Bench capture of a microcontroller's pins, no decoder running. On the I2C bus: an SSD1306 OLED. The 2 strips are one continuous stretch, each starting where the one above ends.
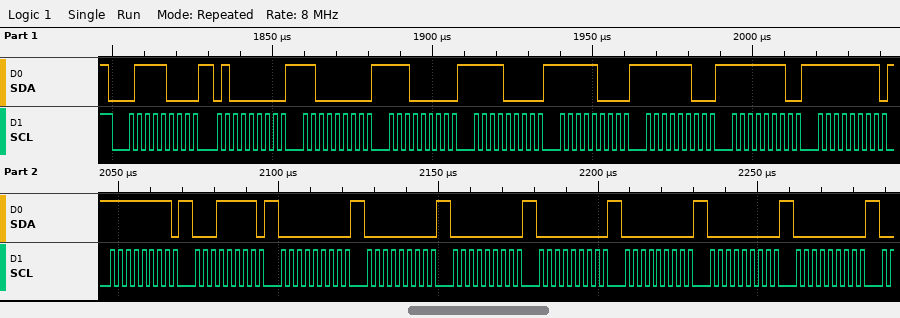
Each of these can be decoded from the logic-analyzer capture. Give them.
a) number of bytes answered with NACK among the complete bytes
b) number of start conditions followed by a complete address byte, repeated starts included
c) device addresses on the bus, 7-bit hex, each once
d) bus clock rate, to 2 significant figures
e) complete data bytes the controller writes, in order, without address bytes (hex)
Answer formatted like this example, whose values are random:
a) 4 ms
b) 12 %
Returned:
a) 0
b) 1
c) 0x3C
d) 400 kHz
e) 40 C0 E0 F0 F8 FC FE FF FF 1F 00 00 00 00 00 00 00
